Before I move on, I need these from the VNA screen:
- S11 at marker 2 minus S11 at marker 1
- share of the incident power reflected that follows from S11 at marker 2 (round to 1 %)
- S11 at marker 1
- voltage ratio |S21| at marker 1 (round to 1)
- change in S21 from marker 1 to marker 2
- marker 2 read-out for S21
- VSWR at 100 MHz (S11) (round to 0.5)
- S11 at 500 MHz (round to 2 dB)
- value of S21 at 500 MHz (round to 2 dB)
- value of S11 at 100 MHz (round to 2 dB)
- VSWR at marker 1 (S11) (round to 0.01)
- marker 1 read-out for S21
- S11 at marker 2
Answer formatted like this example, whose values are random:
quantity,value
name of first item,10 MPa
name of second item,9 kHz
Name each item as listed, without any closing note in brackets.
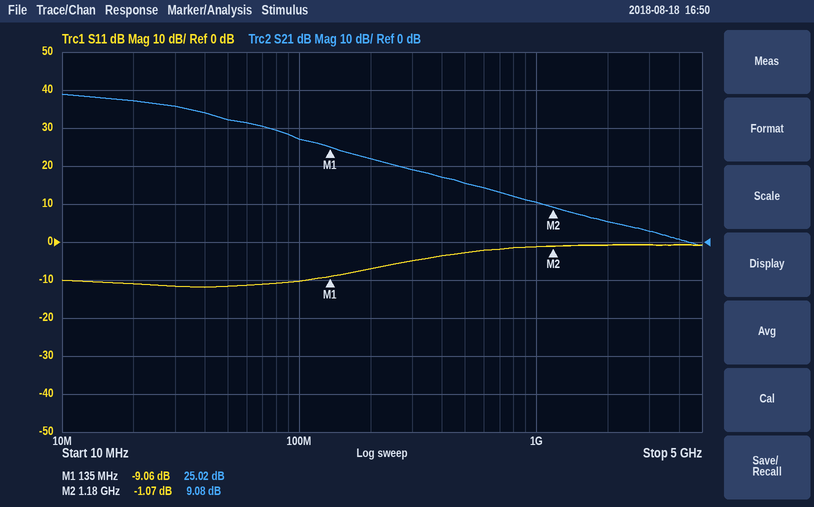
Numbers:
quantity,value
S11 at marker 2 minus S11 at marker 1,7.99 dB
share of the incident power reflected that follows from S11 at marker 2,78 %
S11 at marker 1,-9.06 dB
voltage ratio |S21| at marker 1,18
change in S21 from marker 1 to marker 2,-15.94 dB
marker 2 read-out for S21,9.08 dB
VSWR at 100 MHz (S11),2.0
S11 at 500 MHz,-2 dB
value of S21 at 500 MHz,16 dB
value of S11 at 100 MHz,-10 dB
VSWR at marker 1 (S11),2.09
marker 1 read-out for S21,25.02 dB
S11 at marker 2,-1.07 dB
